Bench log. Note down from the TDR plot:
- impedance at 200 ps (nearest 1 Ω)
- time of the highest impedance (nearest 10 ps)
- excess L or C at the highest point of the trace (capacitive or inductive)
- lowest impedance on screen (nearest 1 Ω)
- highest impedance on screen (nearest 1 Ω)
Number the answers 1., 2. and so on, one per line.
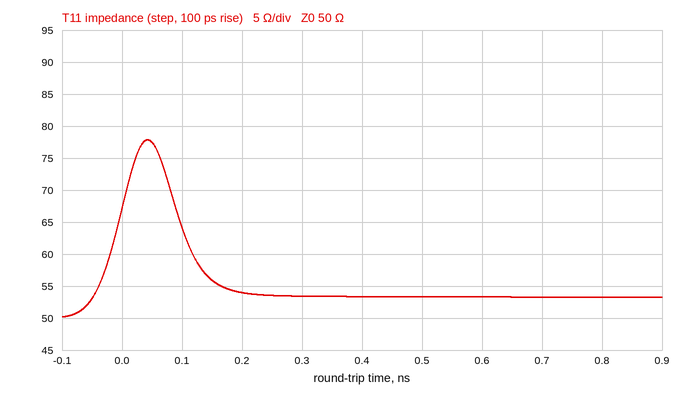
1. 54 Ω
2. 40 ps
3. inductive
4. 50 Ω
5. 78 Ω
